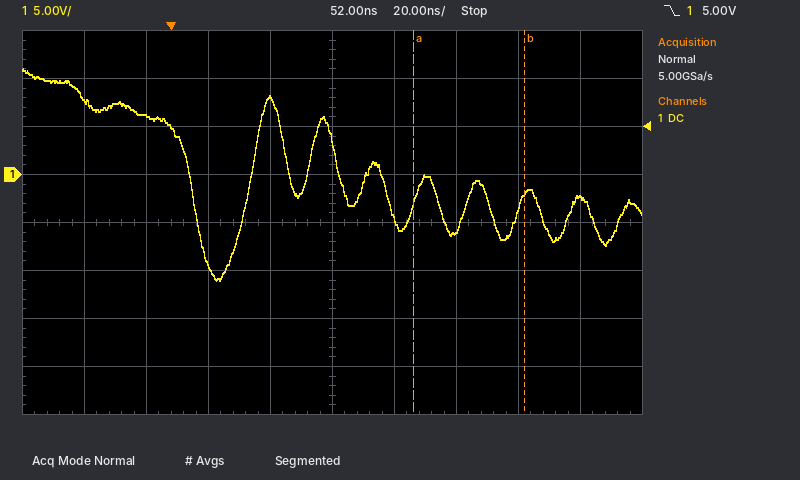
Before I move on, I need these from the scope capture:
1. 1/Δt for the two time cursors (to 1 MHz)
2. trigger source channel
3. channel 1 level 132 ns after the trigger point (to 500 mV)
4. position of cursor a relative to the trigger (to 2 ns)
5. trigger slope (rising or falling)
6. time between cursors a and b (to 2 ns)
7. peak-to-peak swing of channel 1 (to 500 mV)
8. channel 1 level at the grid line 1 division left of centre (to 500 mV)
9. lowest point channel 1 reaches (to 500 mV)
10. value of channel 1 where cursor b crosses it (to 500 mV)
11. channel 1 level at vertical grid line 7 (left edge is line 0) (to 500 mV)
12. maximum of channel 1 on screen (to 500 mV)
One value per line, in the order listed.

28 MHz
channel 1
-2.5 V
+78 ns
falling
36 ns
22.0 V
8.0 V
-11.0 V
-2.0 V
-6.0 V
11.0 V
